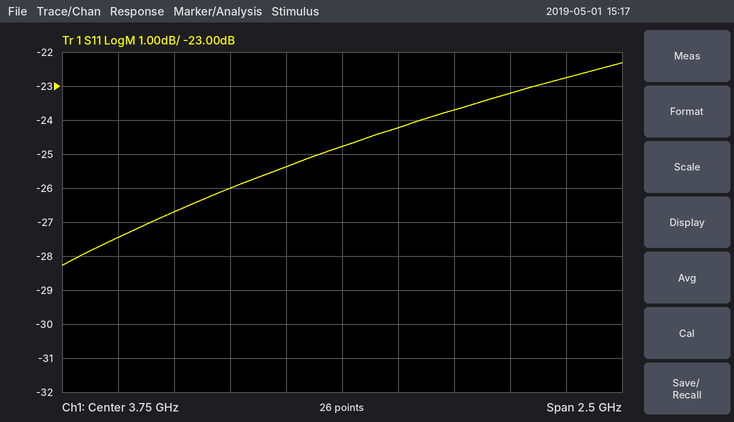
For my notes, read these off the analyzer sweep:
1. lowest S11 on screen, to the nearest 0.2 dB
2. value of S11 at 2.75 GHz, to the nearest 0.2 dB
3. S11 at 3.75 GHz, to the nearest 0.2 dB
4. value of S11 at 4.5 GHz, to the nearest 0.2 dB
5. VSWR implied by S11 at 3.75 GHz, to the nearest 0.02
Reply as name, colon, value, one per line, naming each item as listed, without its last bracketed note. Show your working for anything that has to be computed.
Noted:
lowest S11 on screen, to the nearest 0.2 dB: -28.2 dB
value of S11 at 2.75 GHz, to the nearest 0.2 dB: -27.4 dB
S11 at 3.75 GHz, to the nearest 0.2 dB: -24.8 dB
value of S11 at 4.5 GHz, to the nearest 0.2 dB: -23.2 dB
VSWR implied by S11 at 3.75 GHz, to the nearest 0.02: |Γ| = 10^(-24.8/20) = 0.0575; VSWR = (1 + 0.0575)/(1 − 0.0575) ≈ 1.12
